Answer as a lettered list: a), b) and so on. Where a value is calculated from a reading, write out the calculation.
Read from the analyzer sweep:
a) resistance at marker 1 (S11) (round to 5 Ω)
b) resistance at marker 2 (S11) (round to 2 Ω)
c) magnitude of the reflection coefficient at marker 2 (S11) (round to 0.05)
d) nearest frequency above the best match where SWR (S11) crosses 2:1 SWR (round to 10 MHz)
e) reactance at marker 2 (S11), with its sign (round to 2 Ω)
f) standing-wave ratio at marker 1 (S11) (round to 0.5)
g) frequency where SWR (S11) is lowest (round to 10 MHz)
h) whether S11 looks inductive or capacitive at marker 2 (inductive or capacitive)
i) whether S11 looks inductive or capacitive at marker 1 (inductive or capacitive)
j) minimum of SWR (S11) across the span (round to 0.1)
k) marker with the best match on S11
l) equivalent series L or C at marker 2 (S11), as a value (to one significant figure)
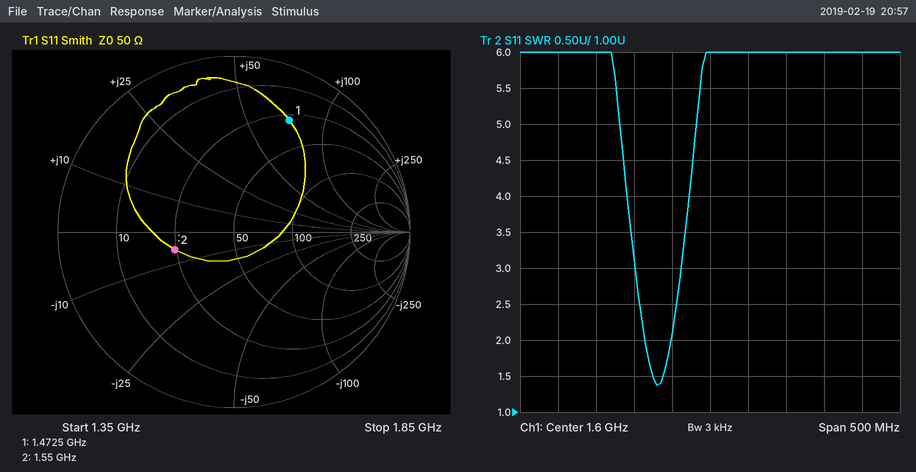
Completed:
a) 30 Ω
b) 24 Ω
c) 0.35
d) 1.55 GHz
e) -6 Ω
f) 6.0
g) 1.53 GHz
h) capacitive
i) inductive
j) 1.4
k) marker 2
l) C = 1/(2π × 1.55 GHz × 6 Ω) ≈ 17.1 pF, so 20 pF to one significant figure
